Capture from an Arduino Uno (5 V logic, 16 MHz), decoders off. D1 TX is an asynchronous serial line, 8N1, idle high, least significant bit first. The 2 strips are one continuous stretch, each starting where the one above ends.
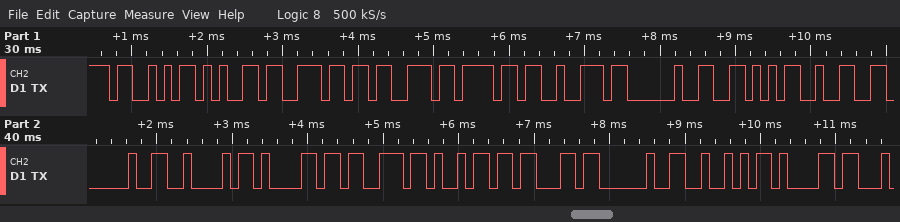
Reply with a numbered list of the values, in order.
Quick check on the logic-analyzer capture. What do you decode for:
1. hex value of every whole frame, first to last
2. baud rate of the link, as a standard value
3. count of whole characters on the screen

1. 53 65 6E 73 6F 72 20 56 32 20 42 61 73 69 63 20 52 61
2. 9600 baud
3. 18
